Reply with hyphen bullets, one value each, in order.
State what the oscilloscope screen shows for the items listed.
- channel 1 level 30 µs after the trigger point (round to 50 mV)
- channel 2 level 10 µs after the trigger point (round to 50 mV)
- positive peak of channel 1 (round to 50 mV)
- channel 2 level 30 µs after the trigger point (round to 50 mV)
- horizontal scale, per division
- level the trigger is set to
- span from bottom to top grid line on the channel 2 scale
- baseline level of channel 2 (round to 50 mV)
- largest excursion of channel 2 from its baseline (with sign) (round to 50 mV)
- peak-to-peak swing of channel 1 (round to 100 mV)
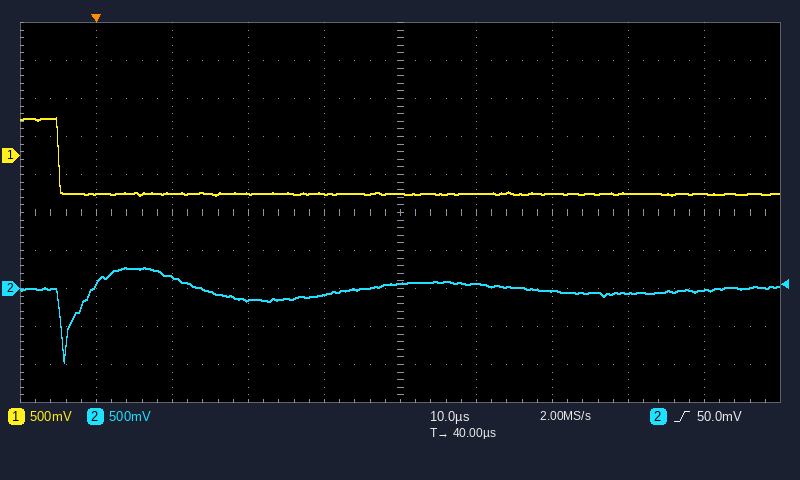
- -500 mV
- 150 mV
- 500 mV
- -100 mV
- 10 µs
- 50.0 mV
- 5 V
- 0 mV
- -950 mV
- 1.00 V
